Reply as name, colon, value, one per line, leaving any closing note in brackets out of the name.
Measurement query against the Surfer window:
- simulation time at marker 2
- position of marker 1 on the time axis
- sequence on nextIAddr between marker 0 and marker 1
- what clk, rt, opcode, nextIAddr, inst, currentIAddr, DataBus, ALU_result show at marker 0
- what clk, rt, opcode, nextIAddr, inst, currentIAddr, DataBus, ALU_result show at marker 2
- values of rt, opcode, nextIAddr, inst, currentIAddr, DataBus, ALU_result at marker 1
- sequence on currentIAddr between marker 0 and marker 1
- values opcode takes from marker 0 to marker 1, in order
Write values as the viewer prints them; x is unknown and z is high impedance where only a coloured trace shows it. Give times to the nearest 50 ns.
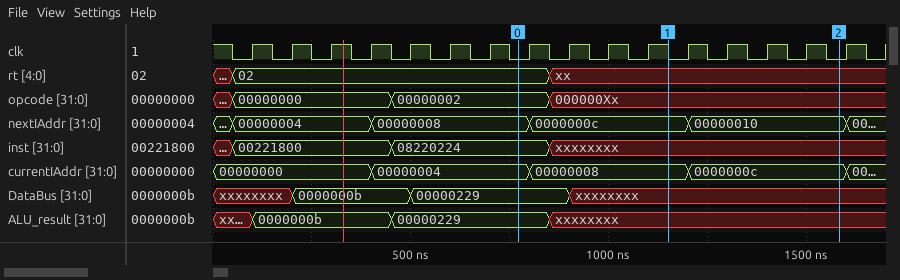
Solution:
simulation time at marker 2: 1600 ns
position of marker 1 on the time axis: 1150 ns
sequence on nextIAddr between marker 0 and marker 1: 00000008, 0000000c
what clk, rt, opcode, nextIAddr, inst, currentIAddr, DataBus, ALU_result show at marker 0: clk=0, rt=02, opcode=00000002, nextIAddr=00000008, inst=08220224, currentIAddr=00000004, DataBus=00000229, ALU_result=00000229
what clk, rt, opcode, nextIAddr, inst, currentIAddr, DataBus, ALU_result show at marker 2: clk=0, rt=xx, opcode=000000Xx, nextIAddr=00000010, inst=xxxxxxxx, currentIAddr=0000000c, DataBus=xxxxxxxx, ALU_result=xxxxxxxx
values of rt, opcode, nextIAddr, inst, currentIAddr, DataBus, ALU_result at marker 1: rt=xx, opcode=000000Xx, nextIAddr=0000000c, inst=xxxxxxxx, currentIAddr=00000008, DataBus=xxxxxxxx, ALU_result=xxxxxxxx
sequence on currentIAddr between marker 0 and marker 1: 00000004, 00000008
values opcode takes from marker 0 to marker 1, in order: 00000002, 000000Xx
